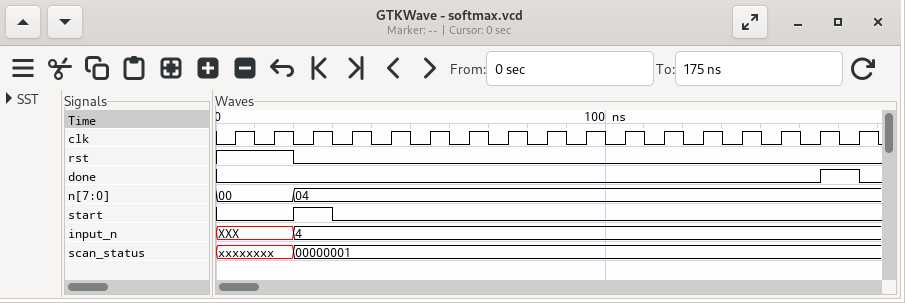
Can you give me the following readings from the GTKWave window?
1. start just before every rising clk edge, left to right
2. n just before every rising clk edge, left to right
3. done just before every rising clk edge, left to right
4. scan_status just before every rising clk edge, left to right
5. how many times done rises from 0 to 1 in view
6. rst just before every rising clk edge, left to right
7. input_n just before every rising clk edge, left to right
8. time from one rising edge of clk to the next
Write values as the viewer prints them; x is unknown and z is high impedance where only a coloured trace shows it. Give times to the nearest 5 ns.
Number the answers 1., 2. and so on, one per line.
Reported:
1. 0 0 1 0 0 0 0 0 0 0 0 0 0 0 0 0 0
2. 00, 00, 04, 04, 04, 04, 04, 04, 04, 04, 04, 04, 04, 04, 04, 04, 04
3. 0 0 0 0 0 0 0 0 0 0 0 0 0 0 0 0 1
4. xxxxxxxx, xxxxxxxx, 00000001, 00000001, 00000001, 00000001, 00000001, 00000001, 00000001, 00000001, 00000001, 00000001, 00000001, 00000001, 00000001, 00000001, 00000001
5. 1
6. 1 1 0 0 0 0 0 0 0 0 0 0 0 0 0 0 0
7. XXX, XXX, 4, 4, 4, 4, 4, 4, 4, 4, 4, 4, 4, 4, 4, 4, 4
8. 10 ns
